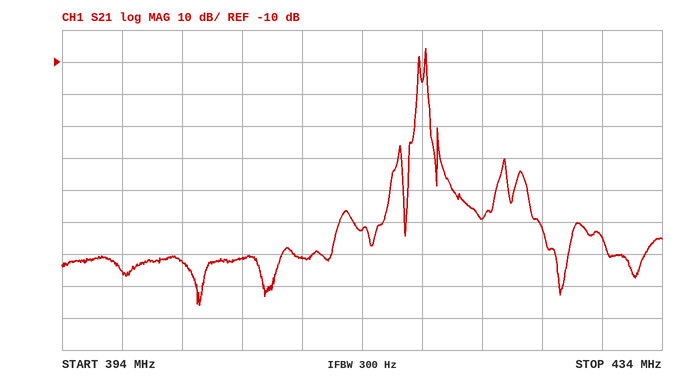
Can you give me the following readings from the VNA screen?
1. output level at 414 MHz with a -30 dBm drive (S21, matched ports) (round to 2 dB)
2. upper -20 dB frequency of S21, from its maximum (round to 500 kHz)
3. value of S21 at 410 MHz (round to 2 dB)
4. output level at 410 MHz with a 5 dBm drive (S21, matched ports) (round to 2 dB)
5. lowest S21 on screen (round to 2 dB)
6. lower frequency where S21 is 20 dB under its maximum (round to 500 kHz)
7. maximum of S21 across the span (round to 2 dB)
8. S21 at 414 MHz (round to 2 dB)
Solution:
-92 dBm
418.5 MHz
-72 dB
-66 dBm
-86 dB
417.5 MHz
-6 dB
-62 dB
